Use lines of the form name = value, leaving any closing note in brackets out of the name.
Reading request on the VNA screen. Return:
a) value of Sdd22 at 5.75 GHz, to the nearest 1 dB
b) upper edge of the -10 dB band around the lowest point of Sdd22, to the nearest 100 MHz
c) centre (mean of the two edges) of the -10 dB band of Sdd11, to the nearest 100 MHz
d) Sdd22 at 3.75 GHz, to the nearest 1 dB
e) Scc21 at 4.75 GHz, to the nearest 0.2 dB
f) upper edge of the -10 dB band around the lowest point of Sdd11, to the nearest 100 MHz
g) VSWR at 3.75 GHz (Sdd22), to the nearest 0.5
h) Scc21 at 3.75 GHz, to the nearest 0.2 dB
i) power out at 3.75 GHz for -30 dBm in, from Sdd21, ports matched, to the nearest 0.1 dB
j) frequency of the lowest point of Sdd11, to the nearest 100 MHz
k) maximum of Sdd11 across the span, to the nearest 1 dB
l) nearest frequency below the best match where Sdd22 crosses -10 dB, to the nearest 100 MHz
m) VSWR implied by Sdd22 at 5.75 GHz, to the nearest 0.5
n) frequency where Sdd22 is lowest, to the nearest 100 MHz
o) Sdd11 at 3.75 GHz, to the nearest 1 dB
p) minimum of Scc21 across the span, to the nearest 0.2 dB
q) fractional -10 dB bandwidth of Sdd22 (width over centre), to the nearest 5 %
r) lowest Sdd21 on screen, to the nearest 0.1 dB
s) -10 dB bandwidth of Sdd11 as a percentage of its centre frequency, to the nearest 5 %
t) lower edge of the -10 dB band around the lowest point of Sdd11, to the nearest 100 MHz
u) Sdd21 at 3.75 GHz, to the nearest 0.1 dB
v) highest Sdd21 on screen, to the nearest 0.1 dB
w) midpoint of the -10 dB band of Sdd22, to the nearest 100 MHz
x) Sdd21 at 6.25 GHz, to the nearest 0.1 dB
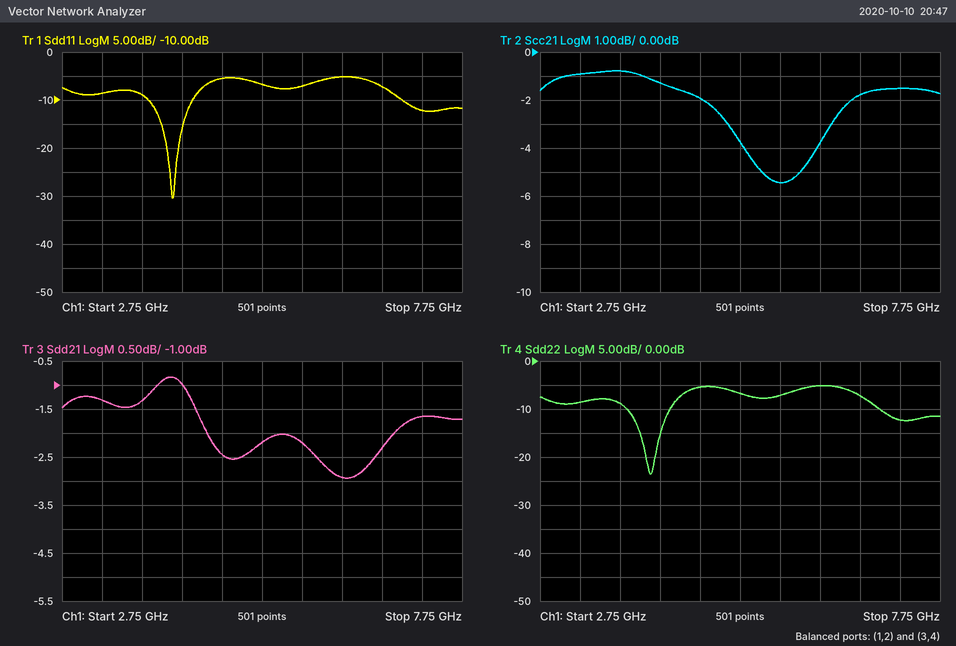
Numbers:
value of Sdd22 at 5.75 GHz, to the nearest 1 dB = -7 dB
upper edge of the -10 dB band around the lowest point of Sdd22, to the nearest 100 MHz = 4.4 GHz
centre (mean of the two edges) of the -10 dB band of Sdd11, to the nearest 100 MHz = 4.1 GHz
Sdd22 at 3.75 GHz, to the nearest 1 dB = -9 dB
Scc21 at 4.75 GHz, to the nearest 0.2 dB = -2.0 dB
upper edge of the -10 dB band around the lowest point of Sdd11, to the nearest 100 MHz = 4.4 GHz
VSWR at 3.75 GHz (Sdd22), to the nearest 0.5 = 2.0
Scc21 at 3.75 GHz, to the nearest 0.2 dB = -0.8 dB
power out at 3.75 GHz for -30 dBm in, from Sdd21, ports matched, to the nearest 0.1 dB = -31.3 dBm
frequency of the lowest point of Sdd11, to the nearest 100 MHz = 4.1 GHz
maximum of Sdd11 across the span, to the nearest 1 dB = -5 dB
nearest frequency below the best match where Sdd22 crosses -10 dB, to the nearest 100 MHz = 3.8 GHz
VSWR implied by Sdd22 at 5.75 GHz, to the nearest 0.5 = 2.5
frequency where Sdd22 is lowest, to the nearest 100 MHz = 4.1 GHz
Sdd11 at 3.75 GHz, to the nearest 1 dB = -9 dB
minimum of Scc21 across the span, to the nearest 0.2 dB = -5.4 dB
fractional -10 dB bandwidth of Sdd22 (width over centre), to the nearest 5 % = 15 %
lowest Sdd21 on screen, to the nearest 0.1 dB = -2.9 dB
-10 dB bandwidth of Sdd11 as a percentage of its centre frequency, to the nearest 5 % = 15 %
lower edge of the -10 dB band around the lowest point of Sdd11, to the nearest 100 MHz = 3.8 GHz
Sdd21 at 3.75 GHz, to the nearest 0.1 dB = -1.3 dB
highest Sdd21 on screen, to the nearest 0.1 dB = -0.8 dB
midpoint of the -10 dB band of Sdd22, to the nearest 100 MHz = 4.1 GHz
Sdd21 at 6.25 GHz, to the nearest 0.1 dB = -2.9 dB
